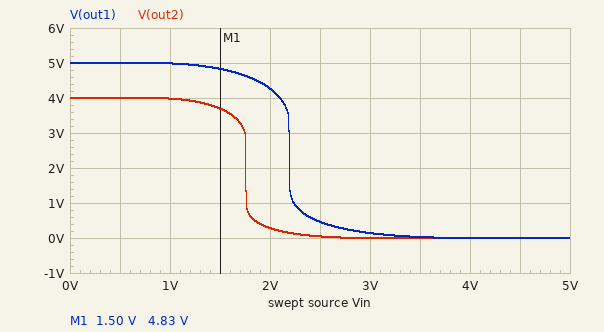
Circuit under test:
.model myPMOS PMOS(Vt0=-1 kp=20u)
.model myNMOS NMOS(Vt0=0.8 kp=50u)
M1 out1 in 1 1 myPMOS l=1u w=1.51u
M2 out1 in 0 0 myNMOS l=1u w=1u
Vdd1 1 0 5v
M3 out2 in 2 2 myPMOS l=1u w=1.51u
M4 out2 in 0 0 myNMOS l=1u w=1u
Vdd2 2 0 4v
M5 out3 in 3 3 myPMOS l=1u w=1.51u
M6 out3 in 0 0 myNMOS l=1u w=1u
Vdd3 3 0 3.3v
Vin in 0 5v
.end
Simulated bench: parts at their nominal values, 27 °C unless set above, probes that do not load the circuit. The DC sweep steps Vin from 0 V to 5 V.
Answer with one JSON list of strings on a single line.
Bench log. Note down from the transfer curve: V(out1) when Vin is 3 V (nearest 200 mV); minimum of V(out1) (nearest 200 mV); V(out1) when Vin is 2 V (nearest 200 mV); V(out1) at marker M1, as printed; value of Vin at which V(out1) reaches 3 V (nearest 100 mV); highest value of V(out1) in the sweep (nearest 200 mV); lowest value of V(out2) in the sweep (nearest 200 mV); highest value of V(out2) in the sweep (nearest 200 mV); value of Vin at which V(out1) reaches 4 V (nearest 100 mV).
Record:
["200 mV", "0 V", "4.2 V", "4.83 V", "2.2 V", "5.0 V", "0 V", "4.0 V", "2.1 V"]
